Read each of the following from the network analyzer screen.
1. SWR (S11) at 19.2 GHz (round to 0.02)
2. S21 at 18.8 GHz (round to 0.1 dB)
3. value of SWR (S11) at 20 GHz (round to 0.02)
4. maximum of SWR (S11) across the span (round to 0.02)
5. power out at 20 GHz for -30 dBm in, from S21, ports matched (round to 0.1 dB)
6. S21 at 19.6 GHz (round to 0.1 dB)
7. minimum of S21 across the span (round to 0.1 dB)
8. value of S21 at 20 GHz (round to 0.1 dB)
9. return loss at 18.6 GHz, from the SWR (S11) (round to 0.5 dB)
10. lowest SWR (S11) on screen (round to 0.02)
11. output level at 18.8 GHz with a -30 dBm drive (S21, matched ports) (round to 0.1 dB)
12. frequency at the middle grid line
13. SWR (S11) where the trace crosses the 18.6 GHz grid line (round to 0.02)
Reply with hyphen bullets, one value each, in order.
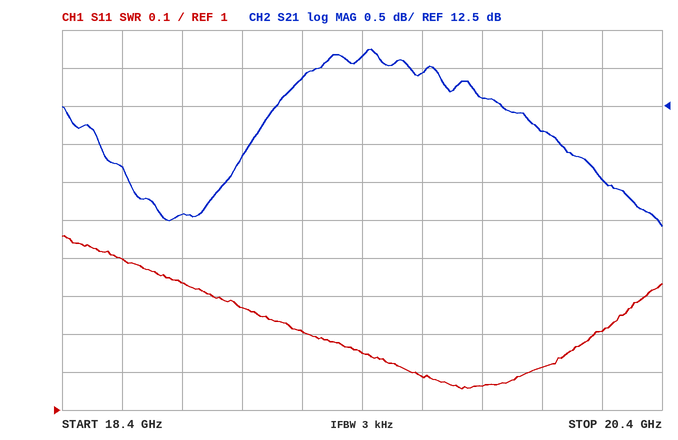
- 1.20
- 11.1 dB
- 1.12
- 1.46
- -17.8 dBm
- 12.9 dB
- 10.9 dB
- 12.2 dB
- 15.5 dB
- 1.06
- -18.9 dBm
- 19.4 GHz
- 1.40
